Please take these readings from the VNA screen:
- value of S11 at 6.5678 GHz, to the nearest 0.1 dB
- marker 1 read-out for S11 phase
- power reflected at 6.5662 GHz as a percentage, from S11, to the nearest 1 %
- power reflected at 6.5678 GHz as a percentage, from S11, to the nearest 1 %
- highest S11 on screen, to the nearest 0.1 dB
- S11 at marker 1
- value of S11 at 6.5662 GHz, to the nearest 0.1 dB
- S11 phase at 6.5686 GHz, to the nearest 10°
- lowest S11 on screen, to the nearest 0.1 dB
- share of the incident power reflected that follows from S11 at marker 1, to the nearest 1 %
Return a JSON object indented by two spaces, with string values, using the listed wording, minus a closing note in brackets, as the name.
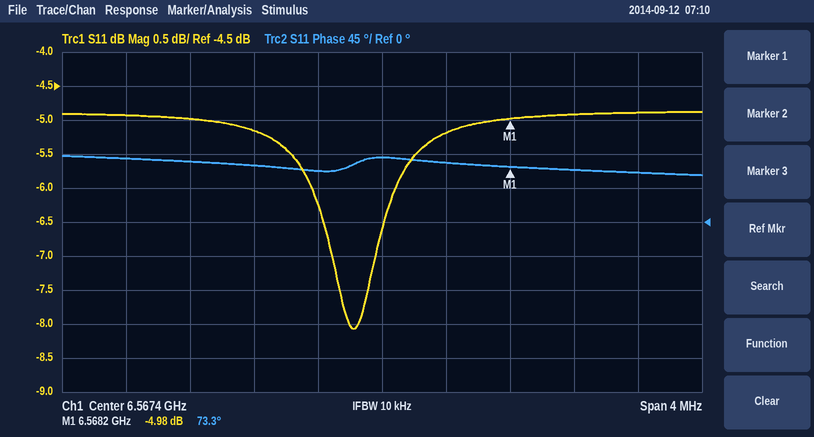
{
  "value of S11 at 6.5678 GHz, to the nearest 0.1 dB": "-5.2 dB",
  "marker 1 read-out for S11 phase": "73.3°",
  "power reflected at 6.5662 GHz as a percentage, from S11, to the nearest 1 %": "32 %",
  "power reflected at 6.5678 GHz as a percentage, from S11, to the nearest 1 %": "30 %",
  "highest S11 on screen, to the nearest 0.1 dB": "-4.9 dB",
  "S11 at marker 1": "-4.98 dB",
  "value of S11 at 6.5662 GHz, to the nearest 0.1 dB": "-5.0 dB",
  "S11 phase at 6.5686 GHz, to the nearest 10°": "70°",
  "lowest S11 on screen, to the nearest 0.1 dB": "-8.1 dB",
  "share of the incident power reflected that follows from S11 at marker 1, to the nearest 1 %": "32 %"
}
